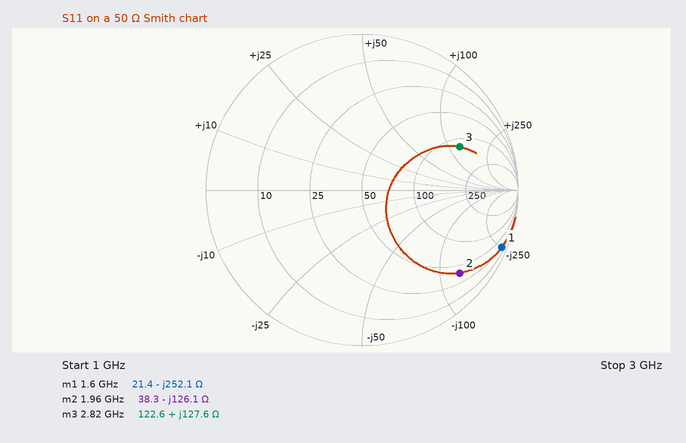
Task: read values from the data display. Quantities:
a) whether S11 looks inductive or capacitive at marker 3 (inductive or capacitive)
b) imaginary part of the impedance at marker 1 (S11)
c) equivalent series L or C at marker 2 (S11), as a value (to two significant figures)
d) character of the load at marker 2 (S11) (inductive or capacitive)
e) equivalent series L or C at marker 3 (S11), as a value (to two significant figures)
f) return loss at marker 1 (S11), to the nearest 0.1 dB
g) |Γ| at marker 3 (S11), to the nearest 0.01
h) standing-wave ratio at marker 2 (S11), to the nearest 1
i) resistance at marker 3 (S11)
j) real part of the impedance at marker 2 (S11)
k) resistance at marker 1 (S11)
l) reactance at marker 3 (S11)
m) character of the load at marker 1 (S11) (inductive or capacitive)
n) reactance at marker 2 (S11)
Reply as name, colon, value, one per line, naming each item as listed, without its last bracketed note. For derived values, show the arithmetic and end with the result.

whether S11 looks inductive or capacitive at marker 3: inductive
imaginary part of the impedance at marker 1: -252.1 Ω
equivalent series L or C at marker 2 (S11), as a value: C = 1/(2π × 1.96 GHz × 126.1 Ω) ≈ 644 fF, so 640 fF to two significant figures
character of the load at marker 2 (S11): capacitive
equivalent series L or C at marker 3 (S11), as a value: L = 127.6 Ω/(2π × 2.82 GHz) ≈ 7.2 nH
return loss at marker 1 (S11), to the nearest 0.1 dB: 0.3 dB
|Γ| at marker 3 (S11), to the nearest 0.01: 0.68
standing-wave ratio at marker 2 (S11), to the nearest 1: 10
resistance at marker 3: 122.6 Ω
real part of the impedance at marker 2: 38.3 Ω
resistance at marker 1: 21.4 Ω
reactance at marker 3: +127.6 Ω
character of the load at marker 1 (S11): capacitive
reactance at marker 2: -126.1 Ω
